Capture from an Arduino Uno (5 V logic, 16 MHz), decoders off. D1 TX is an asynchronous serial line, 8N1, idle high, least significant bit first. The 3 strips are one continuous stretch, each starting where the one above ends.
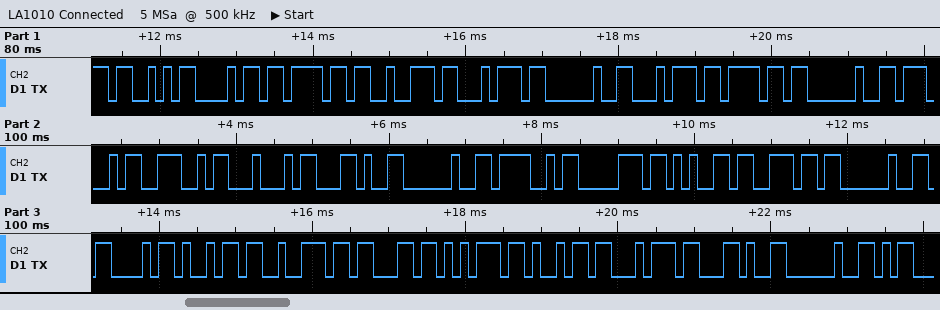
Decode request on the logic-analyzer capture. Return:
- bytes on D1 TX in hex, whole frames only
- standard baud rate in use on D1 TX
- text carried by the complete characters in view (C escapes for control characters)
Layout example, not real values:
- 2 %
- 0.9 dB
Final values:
- 0x53 0x68 0x6F 0x72 0x74 0x20 0x74 0x6F 0x20 0x47 0x4E 0x44 0x2C 0x20 0x4F 0x70 0x65 0x6E 0x20 0x43 0x69 0x72 0x63 0x75 0x69 0x74 0x2C 0x20
- 9600 baud
- "Short to GND, Open Circuit, "
